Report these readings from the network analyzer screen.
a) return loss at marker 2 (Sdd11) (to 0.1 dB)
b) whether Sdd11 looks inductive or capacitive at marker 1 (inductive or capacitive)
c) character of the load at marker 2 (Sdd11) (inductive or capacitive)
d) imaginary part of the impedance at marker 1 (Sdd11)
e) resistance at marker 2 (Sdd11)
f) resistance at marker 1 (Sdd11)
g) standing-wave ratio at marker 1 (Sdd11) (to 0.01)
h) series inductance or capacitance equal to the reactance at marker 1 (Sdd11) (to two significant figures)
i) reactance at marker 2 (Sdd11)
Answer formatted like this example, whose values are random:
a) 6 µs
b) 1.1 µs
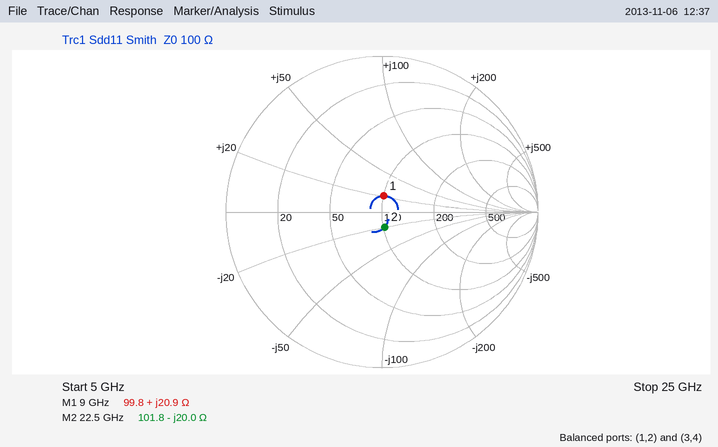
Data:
a) 20.1 dB
b) inductive
c) capacitive
d) +20.9 Ω
e) 101.8 Ω
f) 99.8 Ω
g) 1.23
h) 370 pH
i) -20.0 Ω
